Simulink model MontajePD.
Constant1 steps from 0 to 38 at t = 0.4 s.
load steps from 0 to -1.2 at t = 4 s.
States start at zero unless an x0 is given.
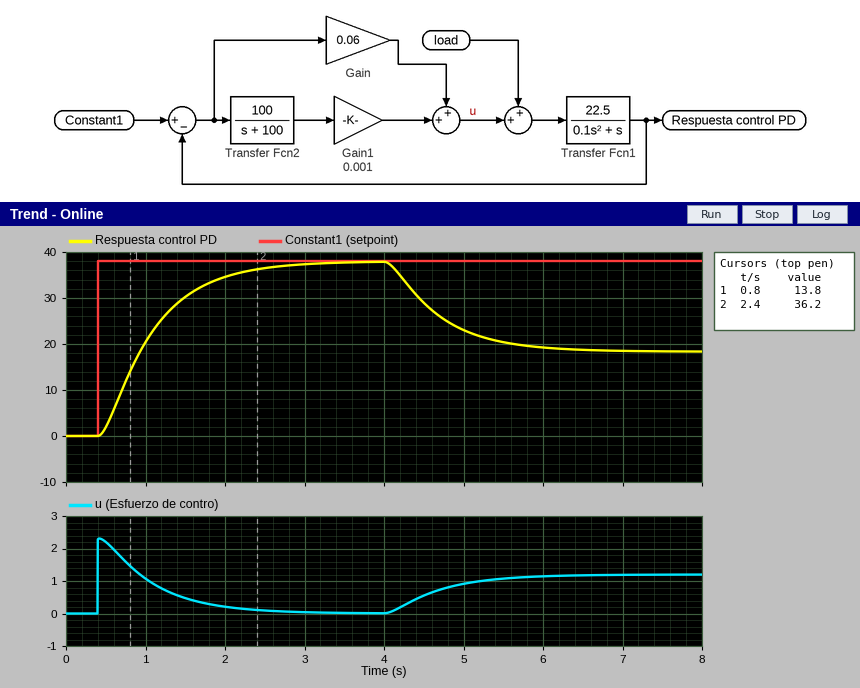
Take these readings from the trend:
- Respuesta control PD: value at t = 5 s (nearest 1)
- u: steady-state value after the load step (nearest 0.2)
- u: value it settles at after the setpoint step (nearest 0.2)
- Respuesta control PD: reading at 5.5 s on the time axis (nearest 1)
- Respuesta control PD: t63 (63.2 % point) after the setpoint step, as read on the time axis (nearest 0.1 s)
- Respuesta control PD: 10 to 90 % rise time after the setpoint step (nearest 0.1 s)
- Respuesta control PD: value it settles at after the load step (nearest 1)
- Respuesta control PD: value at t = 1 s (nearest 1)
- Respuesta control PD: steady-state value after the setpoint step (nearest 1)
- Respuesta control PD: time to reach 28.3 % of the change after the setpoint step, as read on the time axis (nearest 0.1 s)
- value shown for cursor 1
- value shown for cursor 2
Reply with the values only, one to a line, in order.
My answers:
23
1.2
0.0
20
1.1 s
1.4 s
18
20
38
0.7 s
13.8
36.2
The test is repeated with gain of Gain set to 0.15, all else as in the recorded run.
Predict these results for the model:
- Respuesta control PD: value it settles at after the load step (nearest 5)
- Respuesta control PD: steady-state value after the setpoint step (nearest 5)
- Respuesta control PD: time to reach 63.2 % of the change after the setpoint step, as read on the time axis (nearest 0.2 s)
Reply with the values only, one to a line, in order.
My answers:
30
40
0.8 s
